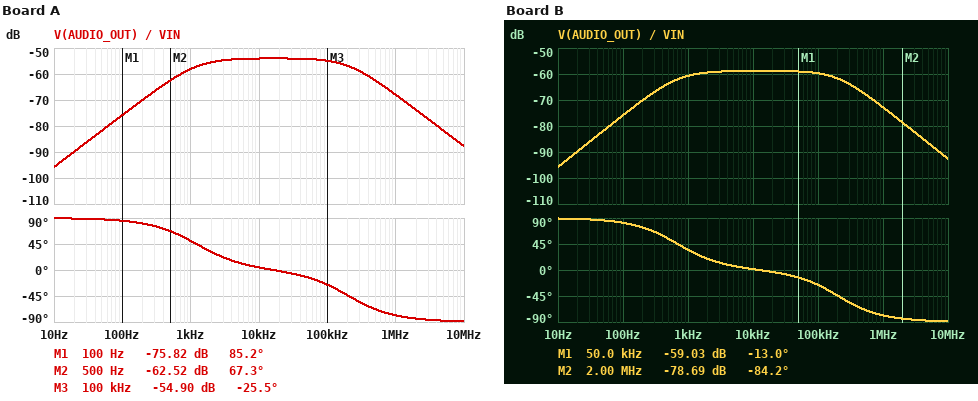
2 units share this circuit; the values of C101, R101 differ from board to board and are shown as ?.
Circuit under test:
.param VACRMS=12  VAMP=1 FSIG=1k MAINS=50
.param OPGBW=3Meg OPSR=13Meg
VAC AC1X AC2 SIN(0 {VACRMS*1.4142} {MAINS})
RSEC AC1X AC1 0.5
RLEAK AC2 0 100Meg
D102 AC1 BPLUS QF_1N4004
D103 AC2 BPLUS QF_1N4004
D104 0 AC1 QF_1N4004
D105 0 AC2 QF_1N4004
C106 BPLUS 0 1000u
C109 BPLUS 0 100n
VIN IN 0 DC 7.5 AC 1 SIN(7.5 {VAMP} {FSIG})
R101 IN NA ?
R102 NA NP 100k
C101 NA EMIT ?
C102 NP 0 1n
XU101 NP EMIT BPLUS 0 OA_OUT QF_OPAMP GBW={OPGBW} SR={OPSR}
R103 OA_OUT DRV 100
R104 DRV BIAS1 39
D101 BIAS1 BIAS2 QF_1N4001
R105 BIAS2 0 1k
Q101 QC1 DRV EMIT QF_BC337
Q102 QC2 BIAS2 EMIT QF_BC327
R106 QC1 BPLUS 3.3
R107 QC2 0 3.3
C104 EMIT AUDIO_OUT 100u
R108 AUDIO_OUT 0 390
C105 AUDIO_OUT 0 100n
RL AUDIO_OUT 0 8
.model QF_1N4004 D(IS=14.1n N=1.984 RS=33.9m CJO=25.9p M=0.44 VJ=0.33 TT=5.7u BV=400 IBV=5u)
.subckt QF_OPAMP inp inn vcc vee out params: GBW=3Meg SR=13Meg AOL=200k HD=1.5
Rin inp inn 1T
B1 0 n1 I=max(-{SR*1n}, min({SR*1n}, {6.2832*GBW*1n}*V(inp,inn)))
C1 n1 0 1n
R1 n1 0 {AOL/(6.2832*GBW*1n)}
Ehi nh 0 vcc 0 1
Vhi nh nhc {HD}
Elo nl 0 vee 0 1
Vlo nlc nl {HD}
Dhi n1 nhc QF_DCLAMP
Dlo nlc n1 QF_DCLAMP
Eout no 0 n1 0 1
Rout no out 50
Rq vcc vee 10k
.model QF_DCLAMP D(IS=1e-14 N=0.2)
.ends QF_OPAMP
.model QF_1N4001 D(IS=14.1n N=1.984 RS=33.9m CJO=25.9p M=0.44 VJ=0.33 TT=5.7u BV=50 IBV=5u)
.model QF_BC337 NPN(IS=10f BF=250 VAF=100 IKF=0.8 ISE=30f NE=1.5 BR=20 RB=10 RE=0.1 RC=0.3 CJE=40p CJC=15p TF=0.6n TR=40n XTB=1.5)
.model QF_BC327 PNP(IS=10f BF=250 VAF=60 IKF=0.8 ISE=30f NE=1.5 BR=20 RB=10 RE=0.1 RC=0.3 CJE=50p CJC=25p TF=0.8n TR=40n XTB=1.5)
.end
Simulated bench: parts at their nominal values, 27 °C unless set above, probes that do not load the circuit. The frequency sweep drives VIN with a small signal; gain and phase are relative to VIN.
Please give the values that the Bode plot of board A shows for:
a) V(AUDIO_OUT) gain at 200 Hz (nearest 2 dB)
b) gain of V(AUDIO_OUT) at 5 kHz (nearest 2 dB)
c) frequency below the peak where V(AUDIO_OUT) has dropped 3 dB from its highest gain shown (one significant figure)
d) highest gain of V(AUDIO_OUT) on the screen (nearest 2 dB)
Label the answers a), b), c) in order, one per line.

a) -70 dB
b) -54 dB
c) 1 kHz
d) -54 dB
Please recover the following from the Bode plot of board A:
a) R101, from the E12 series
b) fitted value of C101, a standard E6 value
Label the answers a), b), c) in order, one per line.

a) 3.9 kΩ
b) 33 nF
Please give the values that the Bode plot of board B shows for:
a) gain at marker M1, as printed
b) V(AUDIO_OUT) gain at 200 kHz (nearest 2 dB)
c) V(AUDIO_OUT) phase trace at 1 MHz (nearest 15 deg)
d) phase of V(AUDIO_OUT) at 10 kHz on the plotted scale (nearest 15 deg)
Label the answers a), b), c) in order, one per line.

a) -59.03 dB
b) -62 dB
c) -75 deg
d) 0 deg
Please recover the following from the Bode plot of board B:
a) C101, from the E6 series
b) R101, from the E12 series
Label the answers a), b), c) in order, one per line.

a) 33 nF
b) 6.8 kΩ
